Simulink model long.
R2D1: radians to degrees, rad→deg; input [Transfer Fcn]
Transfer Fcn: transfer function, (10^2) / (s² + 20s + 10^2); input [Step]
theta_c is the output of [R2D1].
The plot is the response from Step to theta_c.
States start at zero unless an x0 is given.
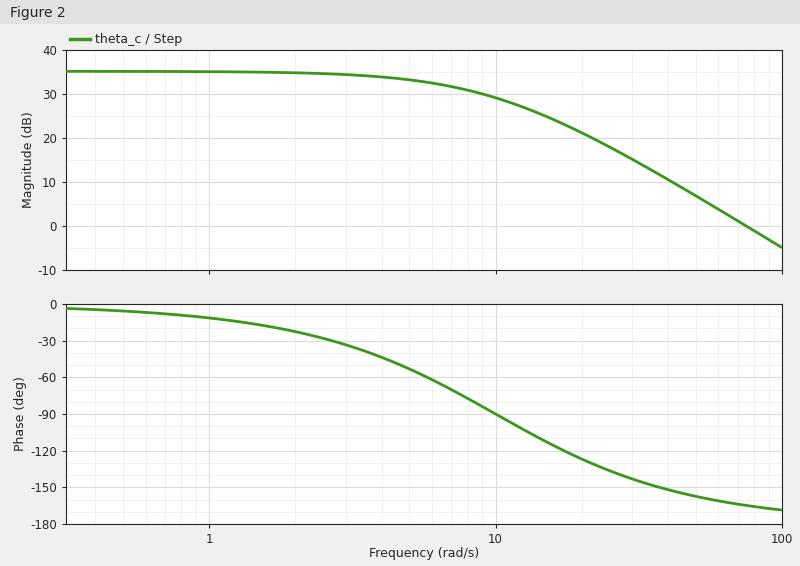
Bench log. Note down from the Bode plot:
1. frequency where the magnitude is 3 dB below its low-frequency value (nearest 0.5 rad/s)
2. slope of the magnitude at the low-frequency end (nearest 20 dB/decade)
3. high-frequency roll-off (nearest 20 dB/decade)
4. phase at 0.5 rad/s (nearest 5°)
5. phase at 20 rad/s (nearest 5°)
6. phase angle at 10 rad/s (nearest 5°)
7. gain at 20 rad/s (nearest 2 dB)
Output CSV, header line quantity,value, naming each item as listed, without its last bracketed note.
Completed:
quantity,value
frequency where the magnitude is 3 dB below its low-frequency value,6.5 rad/s
slope of the magnitude at the low-frequency end,0 dB/decade
high-frequency roll-off,-40 dB/decade
phase at 0.5 rad/s,-5°
phase at 20 rad/s,-125°
phase angle at 10 rad/s,-90°
gain at 20 rad/s,22 dB
